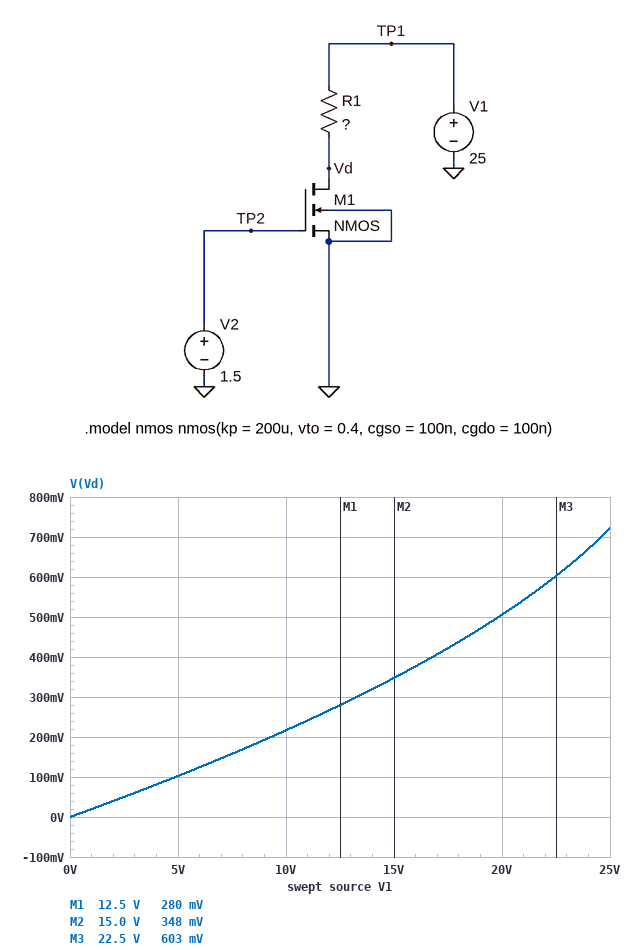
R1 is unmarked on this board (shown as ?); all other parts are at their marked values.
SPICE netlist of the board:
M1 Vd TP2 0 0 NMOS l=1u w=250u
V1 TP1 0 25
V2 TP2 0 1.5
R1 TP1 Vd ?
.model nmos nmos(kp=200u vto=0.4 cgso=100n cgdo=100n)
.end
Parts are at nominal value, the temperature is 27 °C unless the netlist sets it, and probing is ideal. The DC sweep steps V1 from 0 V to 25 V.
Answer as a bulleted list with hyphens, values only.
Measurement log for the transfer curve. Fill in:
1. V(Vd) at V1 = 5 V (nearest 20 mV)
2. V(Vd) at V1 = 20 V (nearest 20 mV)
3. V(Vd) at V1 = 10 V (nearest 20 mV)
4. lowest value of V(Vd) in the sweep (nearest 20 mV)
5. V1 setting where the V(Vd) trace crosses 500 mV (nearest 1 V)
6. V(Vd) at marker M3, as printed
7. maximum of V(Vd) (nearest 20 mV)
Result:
- 100 mV
- 500 mV
- 220 mV
- 0 V
- 20 V
- 603 mV
- 720 mV
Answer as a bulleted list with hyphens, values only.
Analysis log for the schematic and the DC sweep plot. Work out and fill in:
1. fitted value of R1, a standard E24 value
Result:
- 910 Ω
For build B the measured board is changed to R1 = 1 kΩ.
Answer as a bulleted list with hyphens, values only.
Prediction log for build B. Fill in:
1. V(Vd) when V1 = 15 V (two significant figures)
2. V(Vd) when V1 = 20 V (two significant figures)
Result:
- 310 mV
- 450 mV
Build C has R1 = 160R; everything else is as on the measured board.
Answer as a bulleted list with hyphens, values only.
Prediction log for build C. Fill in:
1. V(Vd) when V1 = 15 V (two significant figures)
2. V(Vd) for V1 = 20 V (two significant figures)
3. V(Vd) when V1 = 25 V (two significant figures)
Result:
- 10 V
- 15 V
- 20 V
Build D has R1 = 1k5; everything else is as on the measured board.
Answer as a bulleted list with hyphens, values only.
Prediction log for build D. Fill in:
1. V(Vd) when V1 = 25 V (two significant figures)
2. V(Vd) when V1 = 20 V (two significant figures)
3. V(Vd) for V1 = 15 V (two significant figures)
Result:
- 360 mV
- 270 mV
- 200 mV
